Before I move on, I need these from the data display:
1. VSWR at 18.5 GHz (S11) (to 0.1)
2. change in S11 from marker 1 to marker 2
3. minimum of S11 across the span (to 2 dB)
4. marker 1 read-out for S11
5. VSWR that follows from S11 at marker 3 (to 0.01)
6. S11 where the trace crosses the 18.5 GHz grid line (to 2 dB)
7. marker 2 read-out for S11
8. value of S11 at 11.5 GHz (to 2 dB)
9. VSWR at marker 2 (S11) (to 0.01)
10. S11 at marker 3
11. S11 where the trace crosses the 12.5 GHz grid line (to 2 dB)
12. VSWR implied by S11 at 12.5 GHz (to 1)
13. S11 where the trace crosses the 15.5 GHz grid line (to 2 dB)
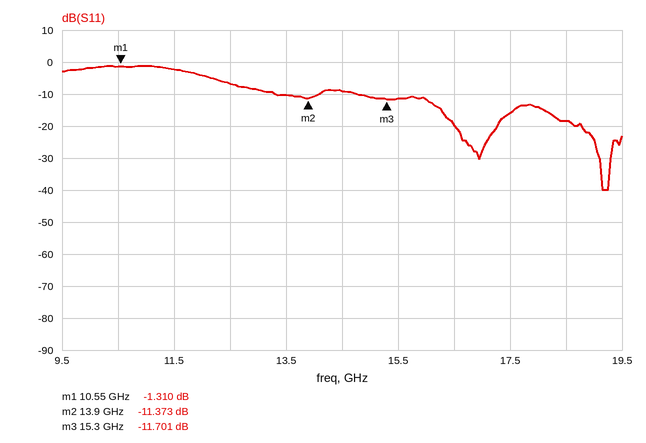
1.3
-10.063 dB
-40 dB
-1.310 dB
1.70
-18 dB
-11.373 dB
-2 dB
1.74
-11.701 dB
-6 dB
3
-12 dB
